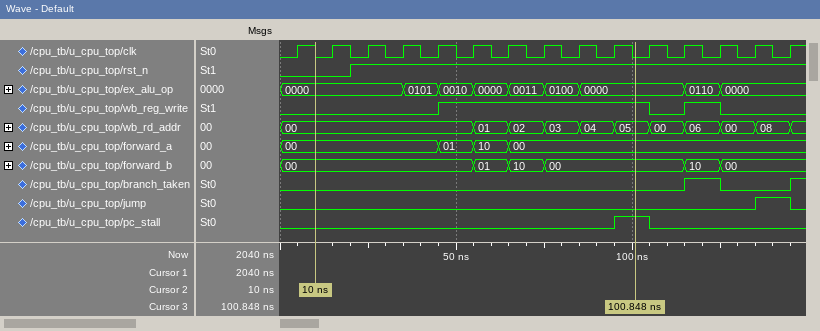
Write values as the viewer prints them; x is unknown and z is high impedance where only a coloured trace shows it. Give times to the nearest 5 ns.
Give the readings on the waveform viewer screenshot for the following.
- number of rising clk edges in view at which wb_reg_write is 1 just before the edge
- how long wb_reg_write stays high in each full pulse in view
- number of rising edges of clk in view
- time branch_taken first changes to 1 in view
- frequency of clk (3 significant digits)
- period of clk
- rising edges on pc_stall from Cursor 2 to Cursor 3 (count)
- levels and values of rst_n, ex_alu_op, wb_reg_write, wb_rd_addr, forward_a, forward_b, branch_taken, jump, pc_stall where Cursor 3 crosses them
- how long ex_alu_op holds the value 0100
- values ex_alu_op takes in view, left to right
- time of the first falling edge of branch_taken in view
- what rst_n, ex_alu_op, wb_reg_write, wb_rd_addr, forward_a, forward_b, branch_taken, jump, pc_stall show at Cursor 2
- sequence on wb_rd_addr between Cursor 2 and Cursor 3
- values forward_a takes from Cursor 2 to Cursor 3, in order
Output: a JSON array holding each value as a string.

["7", "60 ns, 10 ns", "15", "115 ns", "100 MHz", "10 ns", "1", "rst_n=1, ex_alu_op=0000, wb_reg_write=1, wb_rd_addr=05, forward_a=00, forward_b=00, branch_taken=0, jump=0, pc_stall=1", "10 ns", "0000, 0101, 0010, 0000, 0011, 0100, 0000, 0110, 0000", "125 ns", "rst_n=0, ex_alu_op=0000, wb_reg_write=0, wb_rd_addr=00, forward_a=00, forward_b=00, branch_taken=0, jump=0, pc_stall=0", "00, 01, 02, 03, 04, 05", "00, 01, 10, 00"]
